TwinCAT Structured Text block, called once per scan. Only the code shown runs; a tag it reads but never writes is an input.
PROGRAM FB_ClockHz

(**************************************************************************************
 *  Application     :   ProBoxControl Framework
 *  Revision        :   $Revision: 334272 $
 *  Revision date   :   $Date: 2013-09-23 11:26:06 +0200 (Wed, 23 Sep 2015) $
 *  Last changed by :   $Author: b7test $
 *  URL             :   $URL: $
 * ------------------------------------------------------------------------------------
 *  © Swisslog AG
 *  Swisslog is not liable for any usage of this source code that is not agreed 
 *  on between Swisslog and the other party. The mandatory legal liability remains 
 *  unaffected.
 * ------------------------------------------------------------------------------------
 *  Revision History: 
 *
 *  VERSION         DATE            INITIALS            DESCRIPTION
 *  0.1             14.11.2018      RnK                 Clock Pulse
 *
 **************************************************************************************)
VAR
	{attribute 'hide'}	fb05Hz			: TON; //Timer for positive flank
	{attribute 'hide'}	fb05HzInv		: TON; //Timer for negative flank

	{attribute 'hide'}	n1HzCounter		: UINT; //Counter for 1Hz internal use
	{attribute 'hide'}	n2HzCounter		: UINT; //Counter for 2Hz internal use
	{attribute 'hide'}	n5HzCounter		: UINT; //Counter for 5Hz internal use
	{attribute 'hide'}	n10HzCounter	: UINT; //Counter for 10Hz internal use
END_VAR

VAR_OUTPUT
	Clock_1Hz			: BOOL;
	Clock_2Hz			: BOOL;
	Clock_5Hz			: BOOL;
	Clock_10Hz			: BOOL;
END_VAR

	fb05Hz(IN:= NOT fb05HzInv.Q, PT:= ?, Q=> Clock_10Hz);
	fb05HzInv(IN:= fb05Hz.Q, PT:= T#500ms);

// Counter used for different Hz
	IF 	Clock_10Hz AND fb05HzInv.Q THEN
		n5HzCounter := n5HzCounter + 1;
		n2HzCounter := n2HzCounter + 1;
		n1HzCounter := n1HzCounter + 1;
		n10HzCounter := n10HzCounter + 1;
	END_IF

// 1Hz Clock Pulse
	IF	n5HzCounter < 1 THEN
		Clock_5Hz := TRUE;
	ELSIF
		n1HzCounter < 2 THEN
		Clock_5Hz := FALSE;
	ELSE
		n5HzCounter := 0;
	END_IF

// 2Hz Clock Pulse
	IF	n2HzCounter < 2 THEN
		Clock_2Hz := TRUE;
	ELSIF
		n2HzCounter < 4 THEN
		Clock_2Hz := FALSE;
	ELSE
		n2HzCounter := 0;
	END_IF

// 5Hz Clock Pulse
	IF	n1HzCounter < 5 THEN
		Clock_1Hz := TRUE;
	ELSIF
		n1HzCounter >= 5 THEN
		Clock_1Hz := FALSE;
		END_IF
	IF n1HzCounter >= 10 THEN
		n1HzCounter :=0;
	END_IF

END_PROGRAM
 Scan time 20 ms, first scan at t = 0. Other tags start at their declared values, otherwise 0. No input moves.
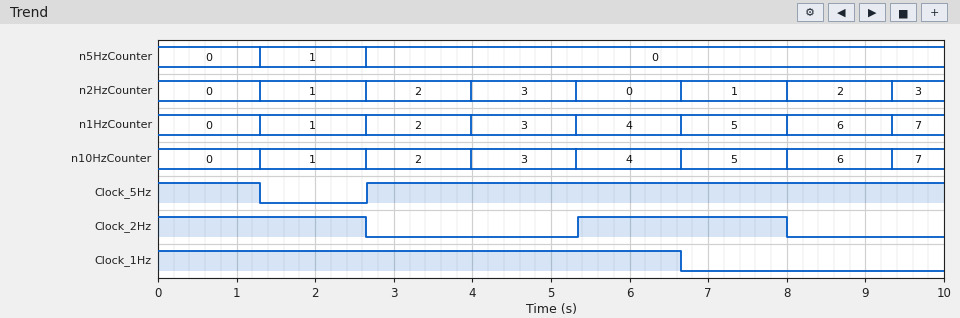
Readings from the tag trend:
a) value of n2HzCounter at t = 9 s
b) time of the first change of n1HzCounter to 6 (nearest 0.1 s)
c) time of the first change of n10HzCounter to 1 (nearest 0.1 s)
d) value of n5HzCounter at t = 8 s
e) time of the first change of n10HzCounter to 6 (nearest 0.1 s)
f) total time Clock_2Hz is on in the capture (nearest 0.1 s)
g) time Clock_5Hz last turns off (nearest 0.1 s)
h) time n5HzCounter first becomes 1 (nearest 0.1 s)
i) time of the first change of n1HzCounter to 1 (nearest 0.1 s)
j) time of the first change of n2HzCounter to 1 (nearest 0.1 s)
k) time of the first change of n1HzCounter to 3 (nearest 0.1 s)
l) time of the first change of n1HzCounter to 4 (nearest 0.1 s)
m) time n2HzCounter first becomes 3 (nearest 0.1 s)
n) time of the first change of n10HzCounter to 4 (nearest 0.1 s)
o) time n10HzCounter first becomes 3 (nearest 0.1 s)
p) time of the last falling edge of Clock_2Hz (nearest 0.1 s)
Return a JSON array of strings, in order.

["2", "8.0 s", "1.3 s", "0", "8.0 s", "5.3 s", "1.3 s", "1.3 s", "1.3 s", "1.3 s", "4.0 s", "5.3 s", "4.0 s", "5.3 s", "4.0 s", "8.0 s"]
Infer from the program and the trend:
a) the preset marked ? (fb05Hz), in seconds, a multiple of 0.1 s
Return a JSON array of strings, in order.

["0.8 s"]
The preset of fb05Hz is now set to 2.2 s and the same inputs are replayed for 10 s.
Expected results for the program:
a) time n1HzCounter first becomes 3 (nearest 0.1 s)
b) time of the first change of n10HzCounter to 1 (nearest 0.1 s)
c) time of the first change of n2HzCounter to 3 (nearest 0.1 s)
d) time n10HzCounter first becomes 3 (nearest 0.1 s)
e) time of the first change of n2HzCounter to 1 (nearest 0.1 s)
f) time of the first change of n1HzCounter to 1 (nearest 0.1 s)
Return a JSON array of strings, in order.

["8.2 s", "2.7 s", "8.2 s", "8.2 s", "2.7 s", "2.7 s"]
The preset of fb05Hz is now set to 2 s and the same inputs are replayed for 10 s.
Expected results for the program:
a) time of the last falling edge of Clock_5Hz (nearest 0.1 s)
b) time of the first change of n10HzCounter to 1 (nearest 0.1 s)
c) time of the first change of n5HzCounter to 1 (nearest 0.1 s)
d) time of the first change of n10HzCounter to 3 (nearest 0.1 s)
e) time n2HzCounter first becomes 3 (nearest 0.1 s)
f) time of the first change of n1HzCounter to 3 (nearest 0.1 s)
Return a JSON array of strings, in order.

["2.5 s", "2.5 s", "2.5 s", "7.6 s", "7.6 s", "7.6 s"]
